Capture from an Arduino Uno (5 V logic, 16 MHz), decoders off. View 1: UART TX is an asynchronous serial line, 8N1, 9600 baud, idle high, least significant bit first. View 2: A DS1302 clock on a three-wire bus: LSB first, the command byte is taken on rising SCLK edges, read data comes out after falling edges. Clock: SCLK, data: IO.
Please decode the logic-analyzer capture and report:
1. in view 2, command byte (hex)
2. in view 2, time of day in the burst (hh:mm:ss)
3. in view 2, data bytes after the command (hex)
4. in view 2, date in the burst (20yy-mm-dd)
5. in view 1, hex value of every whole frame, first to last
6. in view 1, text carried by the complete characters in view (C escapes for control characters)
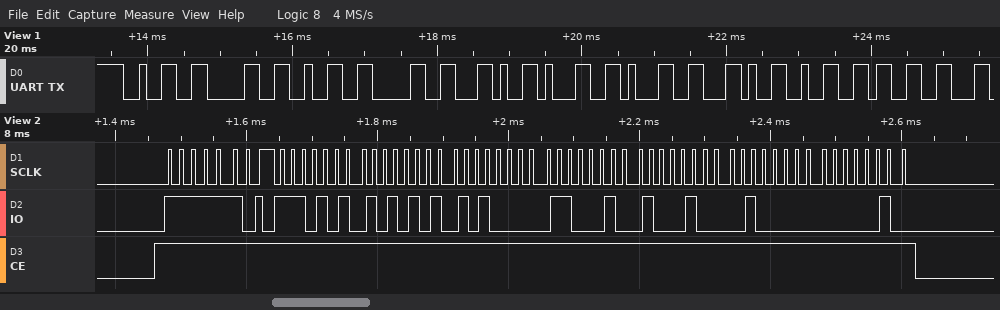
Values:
0xBF
05:55:57
57 55 05 23 11 02 20
2020-11-23
32 30 32 30 2C 31 31 2C 32 33
"2020,11,23"
